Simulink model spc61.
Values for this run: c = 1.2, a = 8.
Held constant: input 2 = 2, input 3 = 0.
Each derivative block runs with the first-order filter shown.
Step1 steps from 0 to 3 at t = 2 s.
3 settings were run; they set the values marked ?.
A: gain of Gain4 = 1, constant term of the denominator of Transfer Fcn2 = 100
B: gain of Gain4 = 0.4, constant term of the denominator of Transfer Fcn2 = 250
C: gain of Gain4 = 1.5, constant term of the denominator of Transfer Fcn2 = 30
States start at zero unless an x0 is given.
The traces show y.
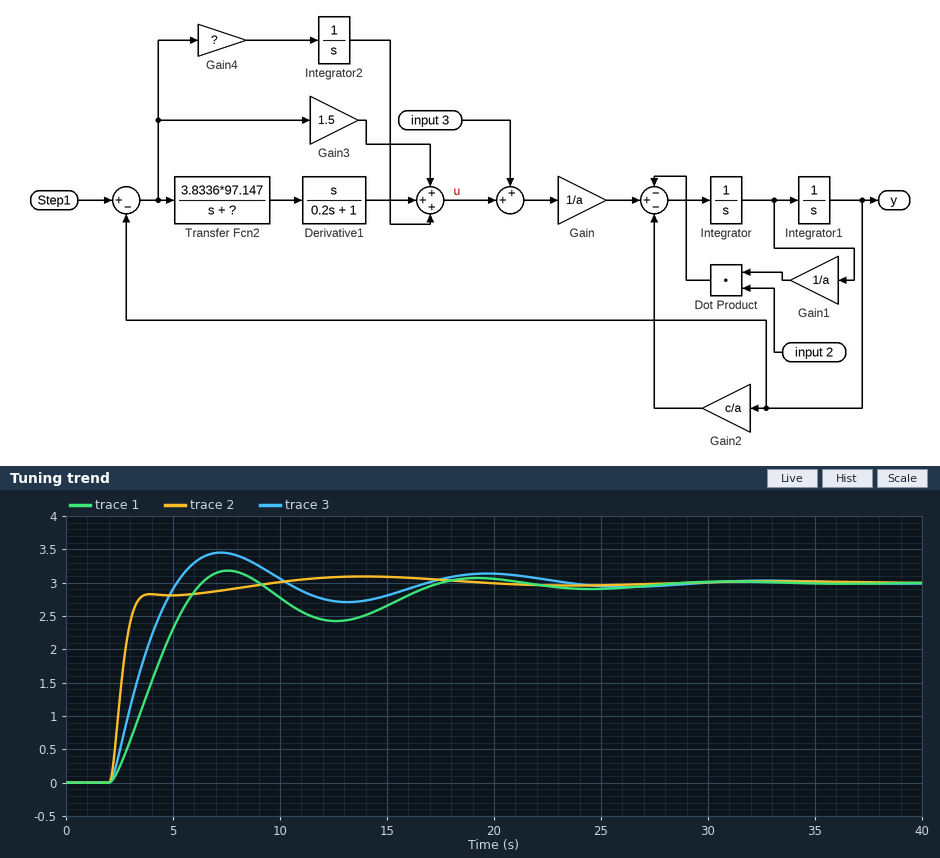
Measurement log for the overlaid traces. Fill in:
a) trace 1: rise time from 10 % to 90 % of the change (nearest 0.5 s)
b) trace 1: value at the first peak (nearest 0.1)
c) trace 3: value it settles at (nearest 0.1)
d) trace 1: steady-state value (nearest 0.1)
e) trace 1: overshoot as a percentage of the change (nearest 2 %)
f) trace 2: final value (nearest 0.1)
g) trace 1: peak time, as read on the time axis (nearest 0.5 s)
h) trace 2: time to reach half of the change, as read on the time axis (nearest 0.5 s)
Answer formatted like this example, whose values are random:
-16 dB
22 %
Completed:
3.0 s
3.2
3.0
3.0
6 %
3.0
7.5 s
2.5 s
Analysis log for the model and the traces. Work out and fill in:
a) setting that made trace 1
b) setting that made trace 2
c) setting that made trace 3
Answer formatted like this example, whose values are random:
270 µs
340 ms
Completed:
B
C
A
